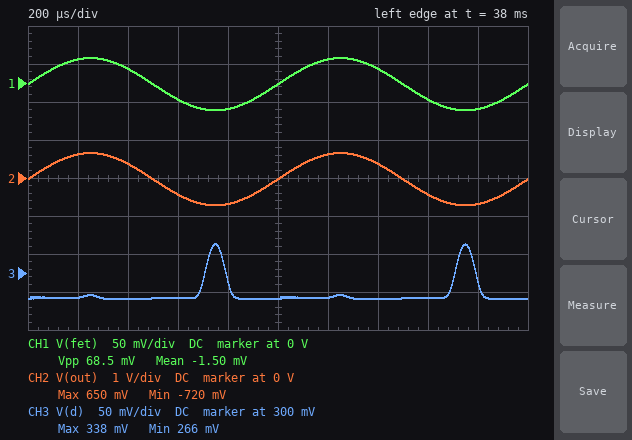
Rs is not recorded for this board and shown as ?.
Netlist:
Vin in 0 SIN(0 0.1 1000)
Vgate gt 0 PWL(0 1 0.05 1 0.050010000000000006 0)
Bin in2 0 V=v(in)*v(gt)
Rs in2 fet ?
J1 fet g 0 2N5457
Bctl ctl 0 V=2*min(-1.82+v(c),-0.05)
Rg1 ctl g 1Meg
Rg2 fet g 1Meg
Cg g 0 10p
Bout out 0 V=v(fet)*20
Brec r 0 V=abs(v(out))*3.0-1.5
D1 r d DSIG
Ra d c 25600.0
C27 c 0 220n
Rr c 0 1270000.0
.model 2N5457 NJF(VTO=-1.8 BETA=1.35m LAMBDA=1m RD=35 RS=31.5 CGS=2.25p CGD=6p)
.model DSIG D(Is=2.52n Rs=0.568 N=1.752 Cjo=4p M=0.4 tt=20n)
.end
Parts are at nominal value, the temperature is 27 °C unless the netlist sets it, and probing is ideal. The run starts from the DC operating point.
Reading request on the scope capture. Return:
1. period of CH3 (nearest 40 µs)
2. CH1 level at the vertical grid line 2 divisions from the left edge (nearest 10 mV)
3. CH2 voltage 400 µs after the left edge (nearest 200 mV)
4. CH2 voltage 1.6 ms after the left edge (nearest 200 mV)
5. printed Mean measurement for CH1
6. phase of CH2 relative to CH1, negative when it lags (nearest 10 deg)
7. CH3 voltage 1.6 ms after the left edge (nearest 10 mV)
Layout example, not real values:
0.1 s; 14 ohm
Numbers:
1.00 ms; 20 mV; 400 mV; -400 mV; -1.50 mV; 0 deg; 270 mV
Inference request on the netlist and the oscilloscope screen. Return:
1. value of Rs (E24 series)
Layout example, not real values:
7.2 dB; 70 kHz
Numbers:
3 kΩ
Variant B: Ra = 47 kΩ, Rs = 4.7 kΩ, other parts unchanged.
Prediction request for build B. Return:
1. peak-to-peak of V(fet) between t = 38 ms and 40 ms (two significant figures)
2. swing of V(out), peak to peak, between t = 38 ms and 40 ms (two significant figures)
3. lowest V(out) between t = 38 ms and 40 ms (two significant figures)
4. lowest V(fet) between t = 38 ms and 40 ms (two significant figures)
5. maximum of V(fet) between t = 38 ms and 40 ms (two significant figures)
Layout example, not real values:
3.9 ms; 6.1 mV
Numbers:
65 mV; 1.3 V; -700 mV; -35 mV; 30 mV
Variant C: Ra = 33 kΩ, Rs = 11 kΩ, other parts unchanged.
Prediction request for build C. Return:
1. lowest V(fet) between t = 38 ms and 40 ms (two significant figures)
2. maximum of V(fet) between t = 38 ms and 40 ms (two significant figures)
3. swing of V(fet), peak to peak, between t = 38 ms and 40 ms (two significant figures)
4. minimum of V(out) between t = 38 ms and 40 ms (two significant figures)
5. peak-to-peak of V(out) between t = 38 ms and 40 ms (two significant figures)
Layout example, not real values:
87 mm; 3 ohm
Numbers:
-32 mV; 22 mV; 54 mV; -640 mV; 1.1 V
